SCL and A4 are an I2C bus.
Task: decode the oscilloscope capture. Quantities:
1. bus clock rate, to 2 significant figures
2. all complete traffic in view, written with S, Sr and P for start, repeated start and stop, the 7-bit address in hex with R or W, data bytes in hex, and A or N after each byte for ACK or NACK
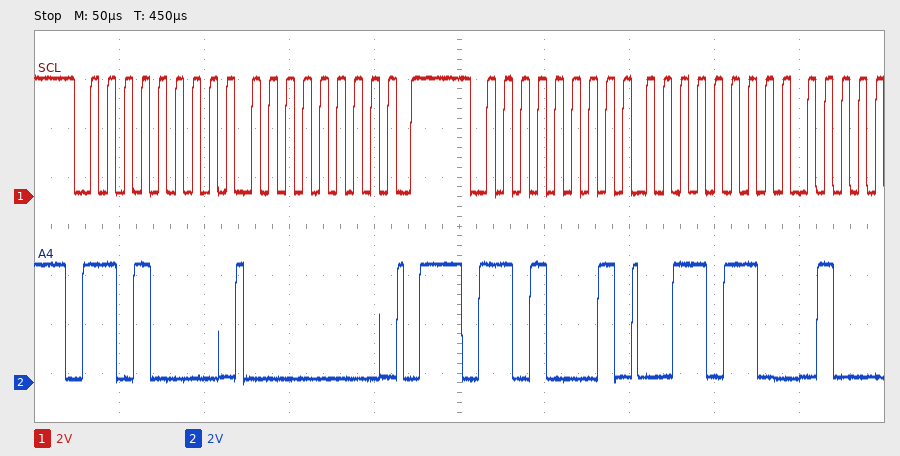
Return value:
100 kHz
S 68W A 00 A P S 68R A 36 A
